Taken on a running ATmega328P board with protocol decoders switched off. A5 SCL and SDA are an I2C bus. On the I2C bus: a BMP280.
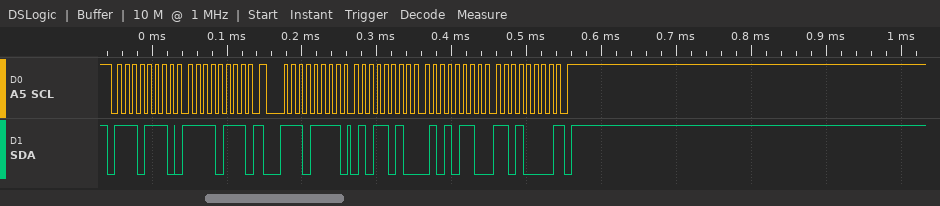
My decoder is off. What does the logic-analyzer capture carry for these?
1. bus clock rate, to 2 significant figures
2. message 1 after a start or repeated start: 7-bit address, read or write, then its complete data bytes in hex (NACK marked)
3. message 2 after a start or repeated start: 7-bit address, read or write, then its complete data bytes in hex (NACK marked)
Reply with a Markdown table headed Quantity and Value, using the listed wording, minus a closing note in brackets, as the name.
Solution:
| Quantity | Value |
|---|---|
| bus clock rate, to 2 significant figures | 100 kHz |
| message 1 after a start or repeated start: 7-bit address, read or write, then its complete data bytes in hex | 0x77 write: F7 |
| message 2 after a start or repeated start: 7-bit address, read or write, then its complete data bytes in hex | 0x77 read: 5A 56 D0 NACK |
